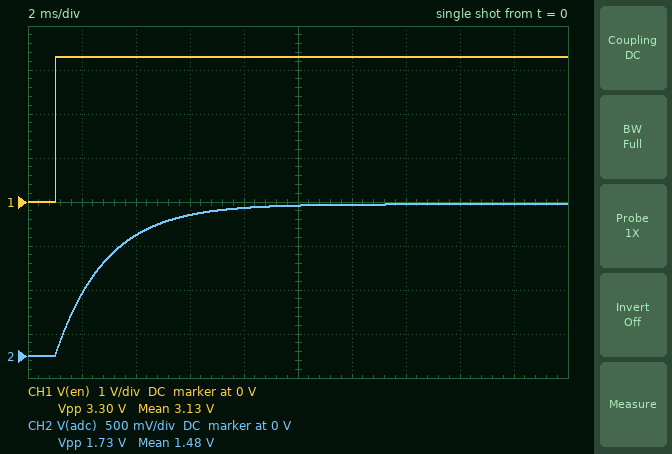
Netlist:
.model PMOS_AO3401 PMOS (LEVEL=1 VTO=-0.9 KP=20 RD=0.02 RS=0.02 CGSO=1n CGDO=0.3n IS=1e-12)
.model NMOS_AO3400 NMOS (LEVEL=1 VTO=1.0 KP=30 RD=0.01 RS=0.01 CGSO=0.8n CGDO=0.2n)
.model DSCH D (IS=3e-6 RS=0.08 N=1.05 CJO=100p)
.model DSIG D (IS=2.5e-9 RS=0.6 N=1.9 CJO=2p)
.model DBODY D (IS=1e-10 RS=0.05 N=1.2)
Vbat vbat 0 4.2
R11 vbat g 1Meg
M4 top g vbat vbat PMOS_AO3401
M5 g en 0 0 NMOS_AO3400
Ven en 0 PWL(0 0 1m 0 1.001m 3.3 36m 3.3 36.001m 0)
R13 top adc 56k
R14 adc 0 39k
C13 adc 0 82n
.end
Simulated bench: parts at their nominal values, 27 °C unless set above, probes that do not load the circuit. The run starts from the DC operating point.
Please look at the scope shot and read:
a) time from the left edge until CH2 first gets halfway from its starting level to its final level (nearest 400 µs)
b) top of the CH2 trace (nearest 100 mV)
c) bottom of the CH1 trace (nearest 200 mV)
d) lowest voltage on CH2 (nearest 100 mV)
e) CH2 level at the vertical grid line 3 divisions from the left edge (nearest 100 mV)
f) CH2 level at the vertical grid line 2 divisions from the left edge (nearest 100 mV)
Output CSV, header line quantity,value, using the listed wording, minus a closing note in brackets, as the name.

quantity,value
time from the left edge until CH2 first gets halfway from its starting level to its final level,2.4 ms
top of the CH2 trace,1.7 V
bottom of the CH1 trace,0 V
lowest voltage on CH2,0 V
CH2 level at the vertical grid line 3 divisions from the left edge,1.6 V
CH2 level at the vertical grid line 2 divisions from the left edge,1.4 V
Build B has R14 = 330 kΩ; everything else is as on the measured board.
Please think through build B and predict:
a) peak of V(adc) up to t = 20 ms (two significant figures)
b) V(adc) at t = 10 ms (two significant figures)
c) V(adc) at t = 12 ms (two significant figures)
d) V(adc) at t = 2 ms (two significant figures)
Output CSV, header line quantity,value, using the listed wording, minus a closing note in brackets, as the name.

quantity,value
peak of V(adc) up to t = 20 ms,3.6 V
V(adc) at t = 10 ms,3.2 V
V(adc) at t = 12 ms,3.4 V
V(adc) at t = 2 ms,810 mV
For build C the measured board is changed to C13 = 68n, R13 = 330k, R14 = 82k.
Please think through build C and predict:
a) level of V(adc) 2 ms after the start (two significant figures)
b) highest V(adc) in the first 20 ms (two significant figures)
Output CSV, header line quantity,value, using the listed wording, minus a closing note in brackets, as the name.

quantity,value
level of V(adc) 2 ms after the start,170 mV
highest V(adc) in the first 20 ms,820 mV
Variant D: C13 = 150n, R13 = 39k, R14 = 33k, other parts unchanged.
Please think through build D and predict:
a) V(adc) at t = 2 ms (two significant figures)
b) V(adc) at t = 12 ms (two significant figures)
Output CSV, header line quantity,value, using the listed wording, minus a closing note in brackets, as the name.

quantity,value
V(adc) at t = 2 ms,600 mV
V(adc) at t = 12 ms,1.9 V
